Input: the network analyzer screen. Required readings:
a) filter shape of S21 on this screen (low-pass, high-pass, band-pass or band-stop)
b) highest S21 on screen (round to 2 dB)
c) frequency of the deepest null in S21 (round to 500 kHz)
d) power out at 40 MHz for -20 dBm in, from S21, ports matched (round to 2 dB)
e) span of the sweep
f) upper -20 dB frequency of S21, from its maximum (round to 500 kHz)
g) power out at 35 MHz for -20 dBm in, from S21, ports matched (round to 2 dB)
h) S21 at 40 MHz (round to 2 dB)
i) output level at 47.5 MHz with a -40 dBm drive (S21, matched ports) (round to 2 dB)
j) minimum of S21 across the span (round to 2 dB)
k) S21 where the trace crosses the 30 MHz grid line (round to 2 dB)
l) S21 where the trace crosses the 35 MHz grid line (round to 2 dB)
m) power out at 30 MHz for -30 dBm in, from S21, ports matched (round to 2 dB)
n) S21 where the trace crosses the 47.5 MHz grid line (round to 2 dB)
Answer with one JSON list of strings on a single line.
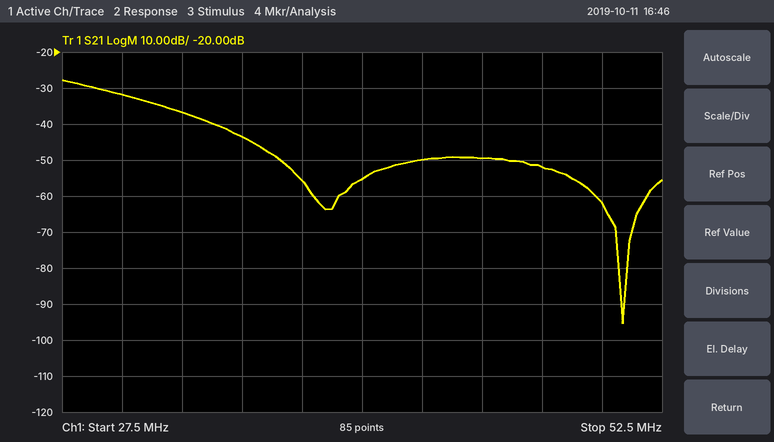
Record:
["low-pass", "-28 dB", "51.0 MHz", "-76 dBm", "25 MHz", "36.0 MHz", "-64 dBm", "-56 dB", "-92 dBm", "-96 dB", "-32 dB", "-44 dB", "-62 dBm", "-52 dB"]
